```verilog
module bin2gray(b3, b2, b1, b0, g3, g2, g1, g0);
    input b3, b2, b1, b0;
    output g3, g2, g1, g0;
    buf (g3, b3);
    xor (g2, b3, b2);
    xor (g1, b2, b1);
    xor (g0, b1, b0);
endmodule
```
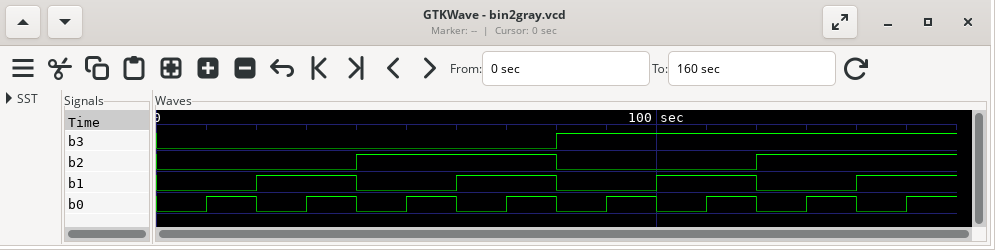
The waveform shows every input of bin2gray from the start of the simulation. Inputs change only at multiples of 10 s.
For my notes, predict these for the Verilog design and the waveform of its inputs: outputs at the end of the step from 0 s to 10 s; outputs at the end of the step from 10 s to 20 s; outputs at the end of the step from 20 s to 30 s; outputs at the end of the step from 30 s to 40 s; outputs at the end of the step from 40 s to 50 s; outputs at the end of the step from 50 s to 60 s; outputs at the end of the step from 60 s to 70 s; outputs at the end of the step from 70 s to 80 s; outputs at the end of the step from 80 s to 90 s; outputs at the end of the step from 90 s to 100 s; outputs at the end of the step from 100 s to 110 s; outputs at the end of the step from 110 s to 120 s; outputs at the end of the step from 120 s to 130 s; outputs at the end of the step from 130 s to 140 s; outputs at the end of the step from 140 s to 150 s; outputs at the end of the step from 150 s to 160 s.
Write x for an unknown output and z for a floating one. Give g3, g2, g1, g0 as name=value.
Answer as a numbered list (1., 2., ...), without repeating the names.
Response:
1. g3=0, g2=0, g1=0, g0=0
2. g3=0, g2=0, g1=0, g0=1
3. g3=0, g2=0, g1=1, g0=1
4. g3=0, g2=0, g1=1, g0=0
5. g3=0, g2=1, g1=1, g0=0
6. g3=0, g2=1, g1=1, g0=1
7. g3=0, g2=1, g1=0, g0=1
8. g3=0, g2=1, g1=0, g0=0
9. g3=1, g2=1, g1=0, g0=0
10. g3=1, g2=1, g1=0, g0=1
11. g3=1, g2=1, g1=1, g0=1
12. g3=1, g2=1, g1=1, g0=0
13. g3=1, g2=0, g1=1, g0=0
14. g3=1, g2=0, g1=1, g0=1
15. g3=1, g2=0, g1=0, g0=1
16. g3=1, g2=0, g1=0, g0=0
